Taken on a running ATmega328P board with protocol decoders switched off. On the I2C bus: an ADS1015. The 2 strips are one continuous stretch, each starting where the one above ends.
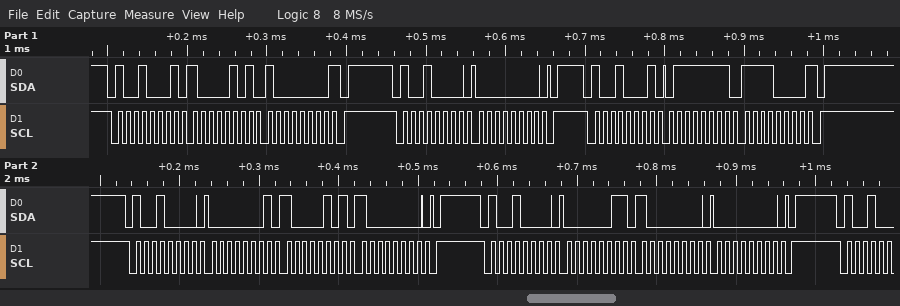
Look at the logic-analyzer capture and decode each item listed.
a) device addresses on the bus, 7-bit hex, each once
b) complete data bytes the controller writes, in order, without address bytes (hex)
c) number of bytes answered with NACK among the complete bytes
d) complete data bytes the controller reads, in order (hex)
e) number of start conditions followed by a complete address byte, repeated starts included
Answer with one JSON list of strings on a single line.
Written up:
["0x48", "00 01 85 80 03 80 00", "2", "85 80 7F F0", "5"]
